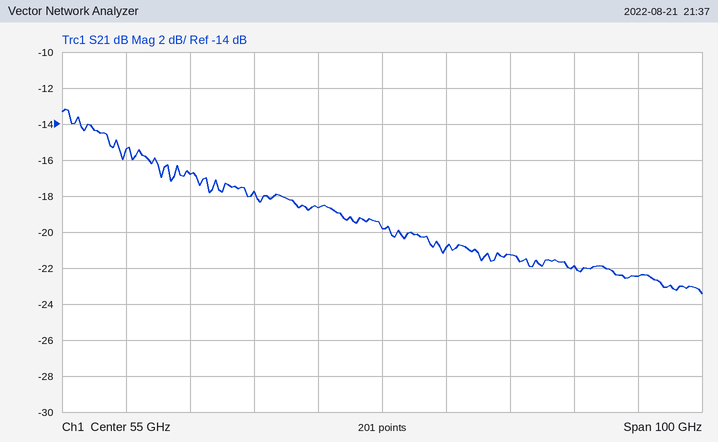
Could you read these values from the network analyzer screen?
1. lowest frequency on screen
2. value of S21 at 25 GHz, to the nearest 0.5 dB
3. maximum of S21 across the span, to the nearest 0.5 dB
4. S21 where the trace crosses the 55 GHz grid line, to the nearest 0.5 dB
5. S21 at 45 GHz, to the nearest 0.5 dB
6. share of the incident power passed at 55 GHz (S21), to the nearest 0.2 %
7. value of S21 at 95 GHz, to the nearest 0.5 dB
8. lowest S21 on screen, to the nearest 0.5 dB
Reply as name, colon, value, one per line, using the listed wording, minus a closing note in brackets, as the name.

lowest frequency on screen: 5 GHz
value of S21 at 25 GHz, to the nearest 0.5 dB: -17.0 dB
maximum of S21 across the span, to the nearest 0.5 dB: -13.0 dB
S21 where the trace crosses the 55 GHz grid line, to the nearest 0.5 dB: -20.0 dB
S21 at 45 GHz, to the nearest 0.5 dB: -18.5 dB
share of the incident power passed at 55 GHz (S21), to the nearest 0.2 %: 1.0 %
value of S21 at 95 GHz, to the nearest 0.5 dB: -22.5 dB
lowest S21 on screen, to the nearest 0.5 dB: -23.5 dB
